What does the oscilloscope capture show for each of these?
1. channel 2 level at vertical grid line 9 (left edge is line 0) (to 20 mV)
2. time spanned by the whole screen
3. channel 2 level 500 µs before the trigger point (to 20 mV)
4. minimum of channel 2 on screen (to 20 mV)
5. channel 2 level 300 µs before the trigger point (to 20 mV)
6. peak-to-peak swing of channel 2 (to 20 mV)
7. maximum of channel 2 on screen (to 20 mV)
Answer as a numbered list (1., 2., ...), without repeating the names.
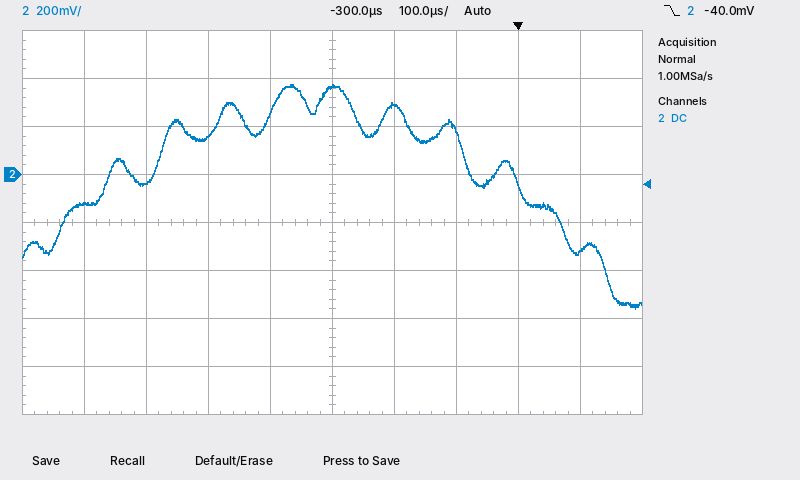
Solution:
1. -320 mV
2. 1 ms
3. 160 mV
4. -560 mV
5. 360 mV
6. 940 mV
7. 380 mV
